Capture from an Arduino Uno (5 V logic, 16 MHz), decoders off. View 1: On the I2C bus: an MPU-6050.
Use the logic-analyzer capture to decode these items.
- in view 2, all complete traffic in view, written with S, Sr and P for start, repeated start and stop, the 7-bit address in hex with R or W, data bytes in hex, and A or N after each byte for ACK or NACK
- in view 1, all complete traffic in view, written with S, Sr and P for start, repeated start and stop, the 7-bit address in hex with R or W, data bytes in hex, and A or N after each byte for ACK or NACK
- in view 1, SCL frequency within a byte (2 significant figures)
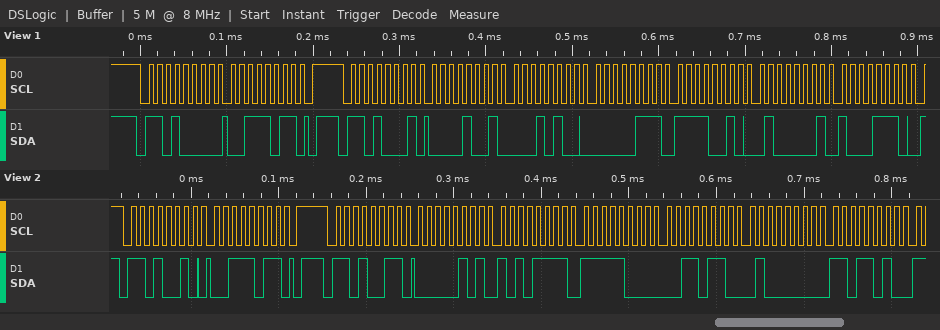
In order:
S 69W A 3B A P S 69R A 05 A AF A F8 A 36 A 40 A DA A
S 68W A 3B A P S 68R A 09 A 14 A 07 A F2 A 41 A 8E A
100 kHz
